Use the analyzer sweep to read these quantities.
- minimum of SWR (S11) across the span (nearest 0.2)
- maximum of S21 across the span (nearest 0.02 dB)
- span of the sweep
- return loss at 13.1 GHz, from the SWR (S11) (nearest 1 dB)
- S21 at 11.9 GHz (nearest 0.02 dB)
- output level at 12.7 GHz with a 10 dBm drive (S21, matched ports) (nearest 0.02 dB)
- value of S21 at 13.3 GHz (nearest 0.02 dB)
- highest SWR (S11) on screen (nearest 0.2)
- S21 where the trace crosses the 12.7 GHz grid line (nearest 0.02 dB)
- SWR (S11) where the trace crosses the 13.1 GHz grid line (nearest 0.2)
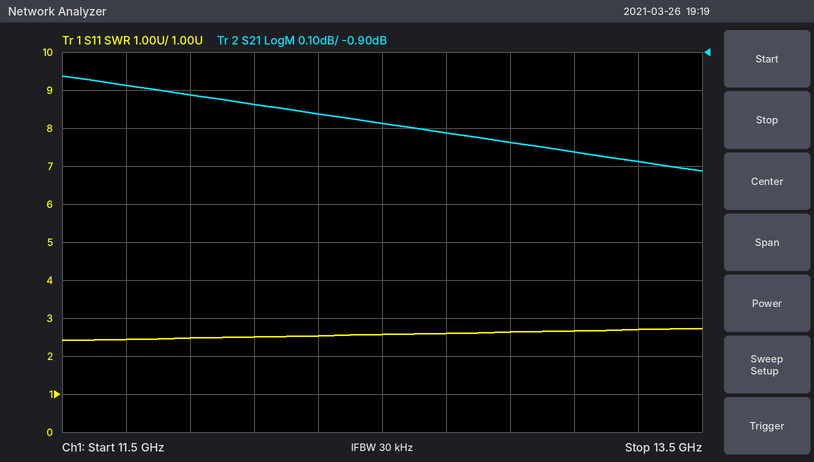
2.4
-0.96 dB
2 GHz
7 dB
-1.02 dB
8.88 dBm
-1.18 dB
2.8
-1.12 dB
2.6
